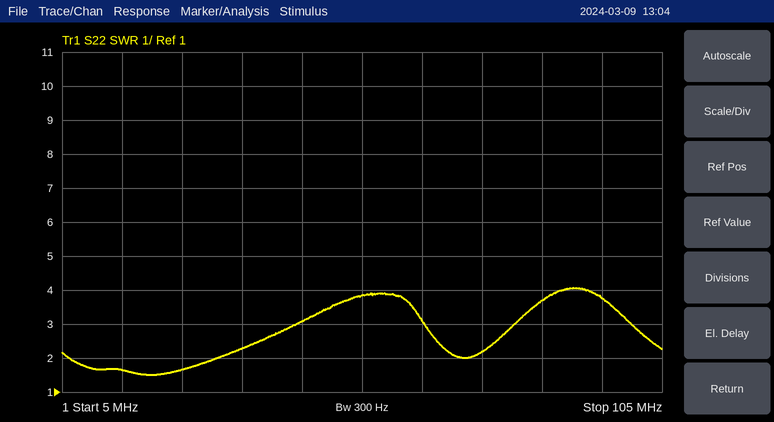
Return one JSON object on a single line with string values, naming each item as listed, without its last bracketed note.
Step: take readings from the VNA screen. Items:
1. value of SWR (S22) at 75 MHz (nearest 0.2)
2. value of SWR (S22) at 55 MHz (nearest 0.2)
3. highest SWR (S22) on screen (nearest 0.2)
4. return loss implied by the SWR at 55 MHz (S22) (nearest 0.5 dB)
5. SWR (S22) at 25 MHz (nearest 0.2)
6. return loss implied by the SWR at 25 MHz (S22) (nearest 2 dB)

{"value of SWR (S22) at 75 MHz": "2.2", "value of SWR (S22) at 55 MHz": "3.8", "highest SWR (S22) on screen": "4.0", "return loss implied by the SWR at 55 MHz (S22)": "4.5 dB", "SWR (S22) at 25 MHz": "1.6", "return loss implied by the SWR at 25 MHz (S22)": "12 dB"}
